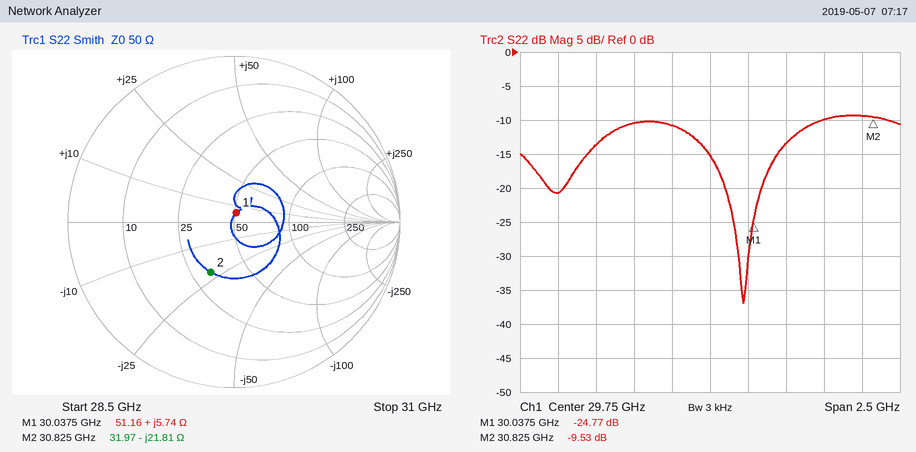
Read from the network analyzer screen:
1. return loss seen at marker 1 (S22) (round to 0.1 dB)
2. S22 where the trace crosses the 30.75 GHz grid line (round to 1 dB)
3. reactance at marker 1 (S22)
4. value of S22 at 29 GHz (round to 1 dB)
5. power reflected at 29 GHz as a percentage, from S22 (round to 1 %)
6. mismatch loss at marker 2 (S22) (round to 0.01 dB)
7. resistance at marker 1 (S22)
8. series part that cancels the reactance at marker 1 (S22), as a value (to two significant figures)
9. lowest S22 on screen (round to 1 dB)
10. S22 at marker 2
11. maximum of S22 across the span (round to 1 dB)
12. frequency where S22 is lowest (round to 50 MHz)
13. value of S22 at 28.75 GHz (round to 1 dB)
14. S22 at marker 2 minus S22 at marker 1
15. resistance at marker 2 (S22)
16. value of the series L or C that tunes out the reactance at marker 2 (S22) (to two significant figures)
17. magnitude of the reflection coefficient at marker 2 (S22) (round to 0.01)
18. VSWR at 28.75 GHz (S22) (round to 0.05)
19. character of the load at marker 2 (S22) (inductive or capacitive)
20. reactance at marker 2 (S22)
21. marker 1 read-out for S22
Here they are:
24.8 dB
-9 dB
+5.74 Ω
-14 dB
4 %
0.51 dB
51.16 Ω
920 fF
-37 dB
-9.53 dB
-9 dB
29.95 GHz
-21 dB
15.24 dB
31.97 Ω
110 pH
0.33
1.20
capacitive
-21.81 Ω
-24.77 dB
